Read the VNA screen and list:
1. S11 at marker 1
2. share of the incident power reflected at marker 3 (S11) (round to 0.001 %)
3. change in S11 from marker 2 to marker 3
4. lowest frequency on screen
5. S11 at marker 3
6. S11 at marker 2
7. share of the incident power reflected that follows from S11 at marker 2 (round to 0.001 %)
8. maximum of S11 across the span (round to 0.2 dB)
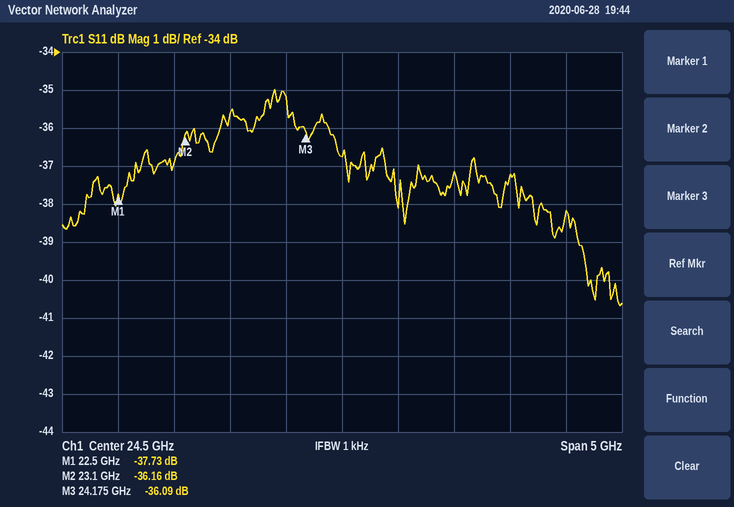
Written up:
-37.73 dB
0.025 %
0.07 dB
22 GHz
-36.09 dB
-36.16 dB
0.024 %
-35.0 dB
